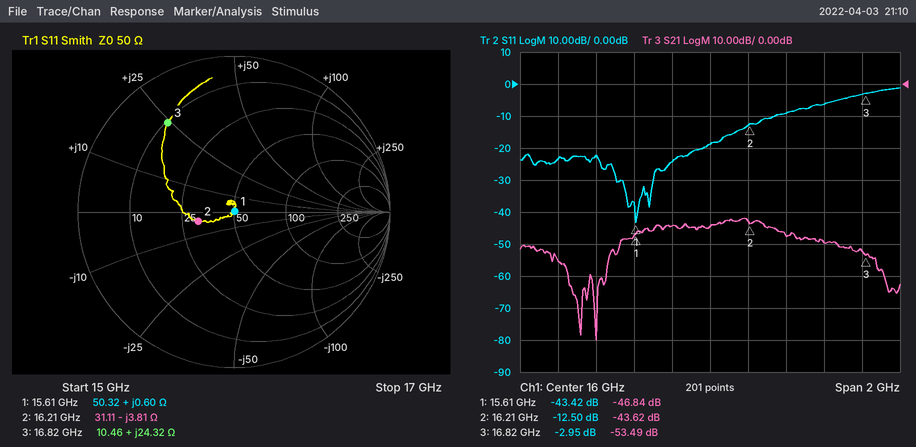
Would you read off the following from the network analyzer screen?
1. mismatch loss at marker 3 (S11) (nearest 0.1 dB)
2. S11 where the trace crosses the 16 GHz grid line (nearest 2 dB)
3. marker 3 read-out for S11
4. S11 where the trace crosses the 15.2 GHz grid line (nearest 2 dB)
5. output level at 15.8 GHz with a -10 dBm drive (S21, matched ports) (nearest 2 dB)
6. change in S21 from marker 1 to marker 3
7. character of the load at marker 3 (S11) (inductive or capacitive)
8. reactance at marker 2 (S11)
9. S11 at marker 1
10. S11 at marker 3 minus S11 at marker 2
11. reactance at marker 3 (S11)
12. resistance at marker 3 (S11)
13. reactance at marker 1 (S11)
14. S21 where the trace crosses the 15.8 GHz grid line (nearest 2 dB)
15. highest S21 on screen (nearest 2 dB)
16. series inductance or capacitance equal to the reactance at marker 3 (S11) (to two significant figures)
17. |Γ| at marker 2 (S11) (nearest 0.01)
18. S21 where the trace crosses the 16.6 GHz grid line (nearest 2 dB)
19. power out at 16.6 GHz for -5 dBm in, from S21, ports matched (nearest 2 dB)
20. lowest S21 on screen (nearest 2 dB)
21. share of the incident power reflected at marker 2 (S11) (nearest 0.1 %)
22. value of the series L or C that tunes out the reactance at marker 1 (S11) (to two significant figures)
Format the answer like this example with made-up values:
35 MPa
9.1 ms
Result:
3.1 dB
-18 dB
-2.95 dB
-24 dB
-54 dBm
-6.65 dB
inductive
-3.81 Ω
-43.42 dB
9.55 dB
+24.32 Ω
10.46 Ω
+0.60 Ω
-44 dB
-42 dB
230 pH
0.24
-50 dB
-54 dBm
-80 dB
5.6 %
17 pF
